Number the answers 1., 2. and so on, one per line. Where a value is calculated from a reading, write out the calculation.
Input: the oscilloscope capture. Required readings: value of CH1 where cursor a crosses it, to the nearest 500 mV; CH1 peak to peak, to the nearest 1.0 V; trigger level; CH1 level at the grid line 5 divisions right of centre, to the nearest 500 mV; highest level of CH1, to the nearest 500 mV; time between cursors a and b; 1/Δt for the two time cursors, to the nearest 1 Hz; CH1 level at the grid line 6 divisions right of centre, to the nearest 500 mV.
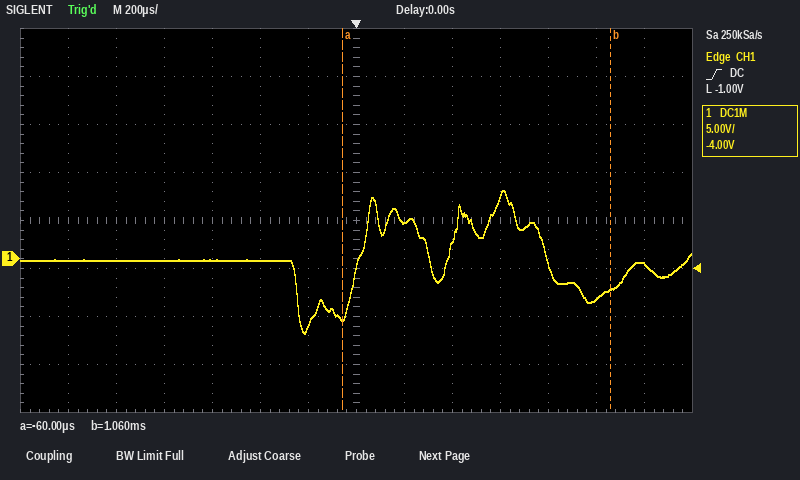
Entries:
1. -6.0 V
2. 15.0 V
3. -1.00 V
4. -4.0 V
5. 7.0 V
6. 1.06 ms − (-60 µs) = 1.12 ms
7. 1 / 1.12 ms ≈ 893 Hz
8. -500 mV
